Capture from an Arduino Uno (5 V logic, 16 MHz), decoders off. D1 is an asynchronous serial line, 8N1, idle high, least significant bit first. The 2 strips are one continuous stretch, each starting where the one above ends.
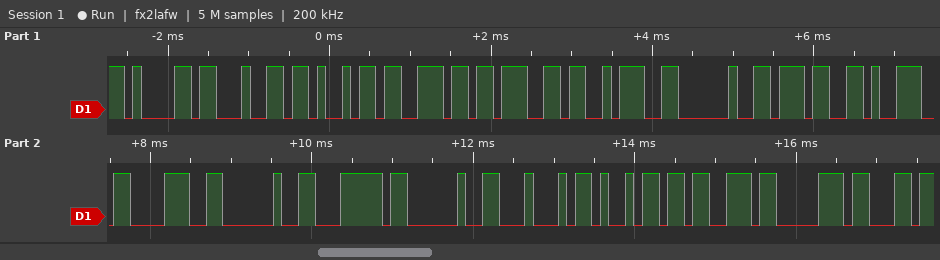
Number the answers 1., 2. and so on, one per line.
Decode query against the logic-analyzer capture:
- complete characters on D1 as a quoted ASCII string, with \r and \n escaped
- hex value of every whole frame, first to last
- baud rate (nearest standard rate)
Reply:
1. "ading: 798 | Disp"
2. 61 64 69 6E 67 3A 20 37 39 38 20 7C 20 44 69 73 70
3. 9600 baud
